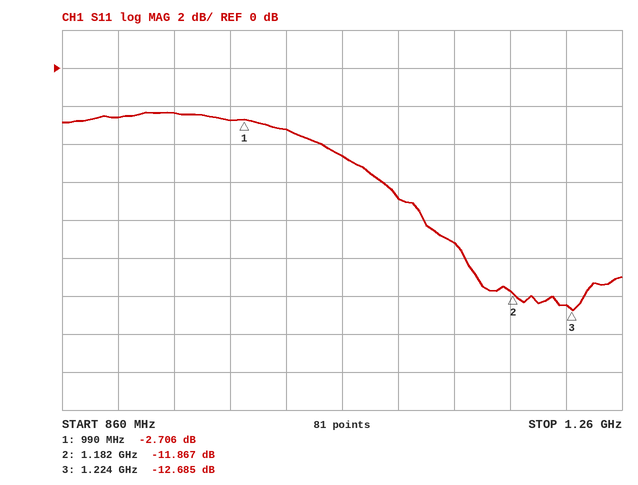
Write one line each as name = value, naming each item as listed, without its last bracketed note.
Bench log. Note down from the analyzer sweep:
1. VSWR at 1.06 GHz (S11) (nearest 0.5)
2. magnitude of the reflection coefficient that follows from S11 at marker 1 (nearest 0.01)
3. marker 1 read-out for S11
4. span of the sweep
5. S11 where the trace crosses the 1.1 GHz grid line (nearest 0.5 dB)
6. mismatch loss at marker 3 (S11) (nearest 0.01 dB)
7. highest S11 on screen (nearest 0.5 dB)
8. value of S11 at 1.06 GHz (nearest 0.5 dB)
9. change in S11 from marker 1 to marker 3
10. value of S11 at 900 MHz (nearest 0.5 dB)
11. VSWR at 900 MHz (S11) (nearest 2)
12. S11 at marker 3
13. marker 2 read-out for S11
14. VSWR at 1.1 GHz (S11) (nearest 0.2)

VSWR at 1.06 GHz (S11) = 4.0
magnitude of the reflection coefficient that follows from S11 at marker 1 = 0.73
marker 1 read-out for S11 = -2.706 dB
span of the sweep = 400 MHz
S11 where the trace crosses the 1.1 GHz grid line = -7.0 dB
mismatch loss at marker 3 (S11) = 0.24 dB
highest S11 on screen = -2.5 dB
value of S11 at 1.06 GHz = -4.5 dB
change in S11 from marker 1 to marker 3 = -9.979 dB
value of S11 at 900 MHz = -2.5 dB
VSWR at 900 MHz (S11) = 6
S11 at marker 3 = -12.685 dB
marker 2 read-out for S11 = -11.867 dB
VSWR at 1.1 GHz (S11) = 2.6
